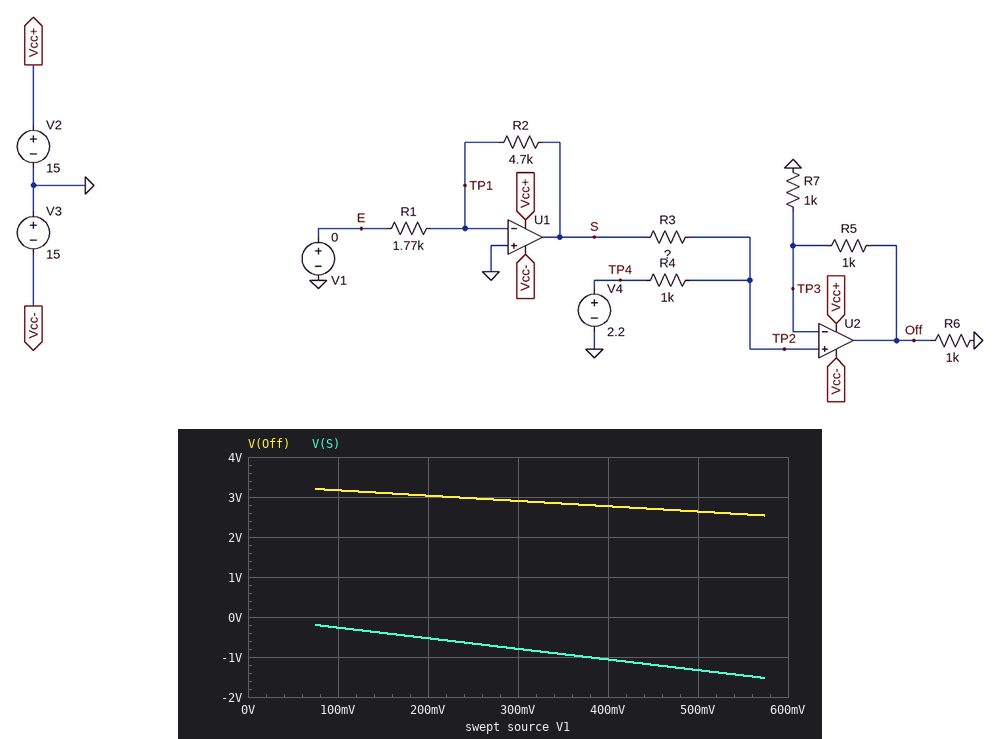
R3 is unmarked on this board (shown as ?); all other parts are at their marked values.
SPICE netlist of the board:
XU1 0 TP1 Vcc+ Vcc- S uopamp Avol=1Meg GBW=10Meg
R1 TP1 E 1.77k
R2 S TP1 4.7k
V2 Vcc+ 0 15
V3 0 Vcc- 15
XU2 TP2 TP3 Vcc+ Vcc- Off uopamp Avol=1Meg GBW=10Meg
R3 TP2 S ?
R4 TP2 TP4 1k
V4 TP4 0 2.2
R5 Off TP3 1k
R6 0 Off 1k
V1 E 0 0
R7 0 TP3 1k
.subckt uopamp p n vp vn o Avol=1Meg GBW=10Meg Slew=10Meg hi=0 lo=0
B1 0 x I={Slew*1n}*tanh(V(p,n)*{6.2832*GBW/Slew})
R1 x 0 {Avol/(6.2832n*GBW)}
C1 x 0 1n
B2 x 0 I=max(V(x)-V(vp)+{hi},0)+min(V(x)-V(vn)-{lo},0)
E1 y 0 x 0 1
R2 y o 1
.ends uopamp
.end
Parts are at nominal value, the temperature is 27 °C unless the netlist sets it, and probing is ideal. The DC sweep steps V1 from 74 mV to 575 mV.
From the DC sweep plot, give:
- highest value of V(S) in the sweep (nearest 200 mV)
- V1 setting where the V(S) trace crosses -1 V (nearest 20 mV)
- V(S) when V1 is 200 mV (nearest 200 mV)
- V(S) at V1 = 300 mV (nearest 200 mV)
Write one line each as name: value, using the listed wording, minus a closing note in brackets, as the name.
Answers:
highest value of V(S) in the sweep: -200 mV
V1 setting where the V(S) trace crosses -1 V: 380 mV
V(S) when V1 is 200 mV: -600 mV
V(S) at V1 = 300 mV: -800 mV
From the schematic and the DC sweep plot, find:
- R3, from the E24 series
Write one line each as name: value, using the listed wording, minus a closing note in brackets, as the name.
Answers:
R3, from the E24 series: 3 kΩ
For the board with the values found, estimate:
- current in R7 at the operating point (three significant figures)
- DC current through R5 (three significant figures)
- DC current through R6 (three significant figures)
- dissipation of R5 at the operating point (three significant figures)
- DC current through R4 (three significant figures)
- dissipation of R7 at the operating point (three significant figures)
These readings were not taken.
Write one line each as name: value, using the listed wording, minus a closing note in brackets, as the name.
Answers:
current in R7 at the operating point: 1.65 mA
DC current through R5: 1.65 mA
DC current through R6: 3.30 mA
dissipation of R5 at the operating point: 2.72 mW
DC current through R4: 550 µA
dissipation of R7 at the operating point: 2.72 mW
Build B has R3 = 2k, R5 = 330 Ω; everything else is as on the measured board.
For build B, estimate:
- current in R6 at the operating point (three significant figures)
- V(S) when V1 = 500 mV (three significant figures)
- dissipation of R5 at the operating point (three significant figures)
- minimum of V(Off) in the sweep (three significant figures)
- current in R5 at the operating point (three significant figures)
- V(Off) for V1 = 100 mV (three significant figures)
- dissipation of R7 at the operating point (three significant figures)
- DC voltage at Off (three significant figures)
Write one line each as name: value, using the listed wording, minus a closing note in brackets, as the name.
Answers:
current in R6 at the operating point: 1.95 mA
V(S) when V1 = 500 mV: -1.33 V
dissipation of R5 at the operating point: 710 µW
minimum of V(Off) in the sweep: 1.27 V
current in R5 at the operating point: 1.47 mA
V(Off) for V1 = 100 mV: 1.83 V
dissipation of R7 at the operating point: 2.15 mW
DC voltage at Off: 1.95 V
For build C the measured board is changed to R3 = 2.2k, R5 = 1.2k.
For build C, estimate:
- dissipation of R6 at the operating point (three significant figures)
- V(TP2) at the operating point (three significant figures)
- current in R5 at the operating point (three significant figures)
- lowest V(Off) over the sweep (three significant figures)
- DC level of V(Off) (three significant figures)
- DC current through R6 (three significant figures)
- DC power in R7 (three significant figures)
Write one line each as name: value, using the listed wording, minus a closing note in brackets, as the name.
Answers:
dissipation of R6 at the operating point: 11.1 mW
V(TP2) at the operating point: 1.51 V
current in R5 at the operating point: 1.51 mA
lowest V(Off) over the sweep: 2.28 V
DC level of V(Off): 3.33 V
DC current through R6: 3.33 mA
DC power in R7: 2.29 mW
